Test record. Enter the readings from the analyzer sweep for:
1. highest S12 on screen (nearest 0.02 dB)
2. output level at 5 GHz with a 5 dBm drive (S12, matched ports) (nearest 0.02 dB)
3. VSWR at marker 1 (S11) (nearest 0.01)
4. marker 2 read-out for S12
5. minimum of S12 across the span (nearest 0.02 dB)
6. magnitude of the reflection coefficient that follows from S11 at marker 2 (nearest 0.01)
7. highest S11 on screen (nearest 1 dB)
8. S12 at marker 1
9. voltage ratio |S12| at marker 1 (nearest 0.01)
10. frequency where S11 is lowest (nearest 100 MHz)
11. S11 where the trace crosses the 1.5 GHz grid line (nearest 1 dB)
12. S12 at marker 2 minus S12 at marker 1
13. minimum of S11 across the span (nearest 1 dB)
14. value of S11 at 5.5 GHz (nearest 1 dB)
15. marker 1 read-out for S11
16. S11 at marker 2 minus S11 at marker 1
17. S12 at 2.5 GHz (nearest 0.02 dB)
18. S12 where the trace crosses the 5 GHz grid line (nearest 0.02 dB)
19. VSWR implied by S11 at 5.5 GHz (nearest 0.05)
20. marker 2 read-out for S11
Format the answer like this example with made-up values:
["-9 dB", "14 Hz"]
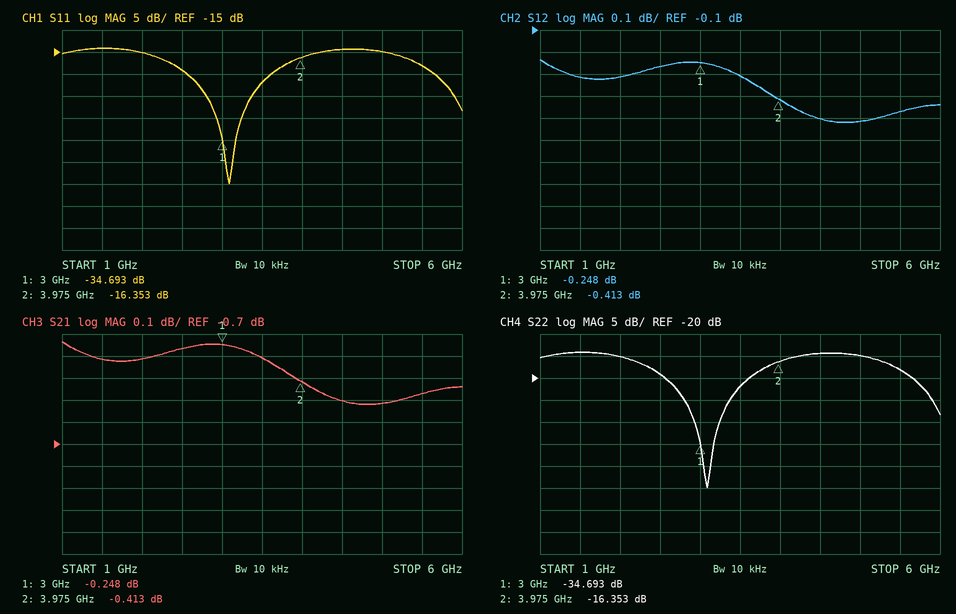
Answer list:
["-0.24 dB", "4.48 dBm", "1.04", "-0.413 dB", "-0.52 dB", "0.15", "-14 dB", "-0.248 dB", "0.97", "3.1 GHz", "-14 dB", "-0.165 dB", "-45 dB", "-18 dB", "-34.693 dB", "18.340 dB", "-0.26 dB", "-0.52 dB", "1.30", "-16.353 dB"]
